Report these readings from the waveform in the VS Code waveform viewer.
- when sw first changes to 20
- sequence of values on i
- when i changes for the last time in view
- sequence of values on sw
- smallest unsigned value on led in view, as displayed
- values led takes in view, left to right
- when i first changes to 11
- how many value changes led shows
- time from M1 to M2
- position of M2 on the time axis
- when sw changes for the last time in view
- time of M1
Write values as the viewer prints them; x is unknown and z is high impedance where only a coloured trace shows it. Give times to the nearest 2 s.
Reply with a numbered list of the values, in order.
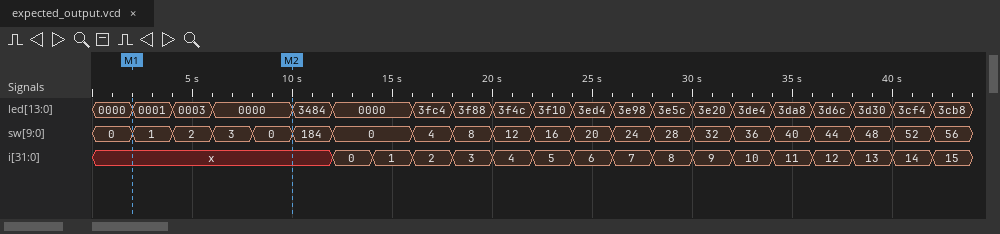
1. 24 s
2. x, 0, 1, 2, 3, 4, 5, 6, 7, 8, 9, 10, 11, 12, 13, 14, 15
3. 42 s
4. 0, 1, 2, 3, 0, 184, 0, 4, 8, 12, 16, 20, 24, 28, 32, 36, 40, 44, 48, 52, 56
5. 0000
6. 0000, 0001, 0003, 0000, 3484, 0000, 3fc4, 3f88, 3f4c, 3f10, 3ed4, 3e98, 3e5c, 3e20, 3de4, 3da8, 3d6c, 3d30, 3cf4, 3cb8
7. 34 s
8. 19
9. 8 s
10. 10 s
11. 42 s
12. 2 s
